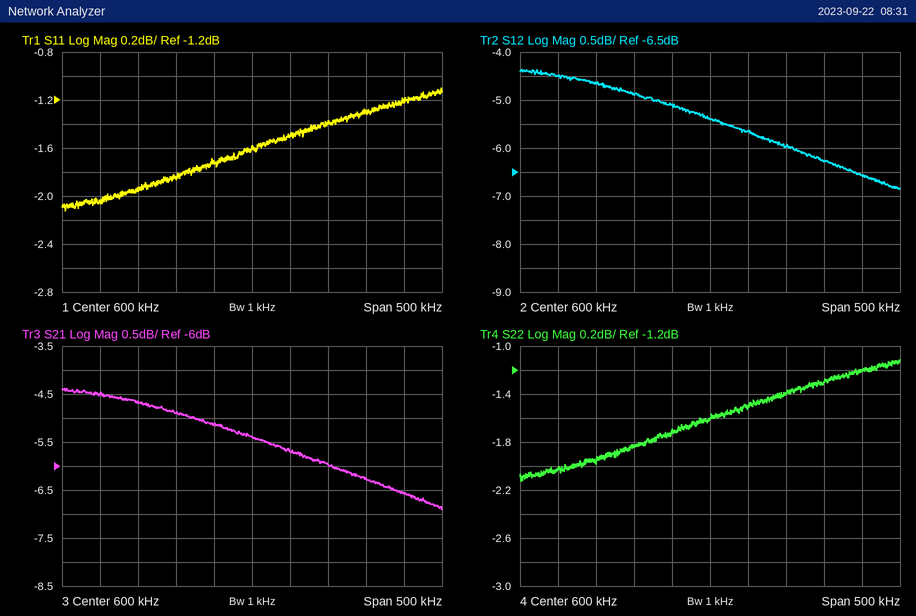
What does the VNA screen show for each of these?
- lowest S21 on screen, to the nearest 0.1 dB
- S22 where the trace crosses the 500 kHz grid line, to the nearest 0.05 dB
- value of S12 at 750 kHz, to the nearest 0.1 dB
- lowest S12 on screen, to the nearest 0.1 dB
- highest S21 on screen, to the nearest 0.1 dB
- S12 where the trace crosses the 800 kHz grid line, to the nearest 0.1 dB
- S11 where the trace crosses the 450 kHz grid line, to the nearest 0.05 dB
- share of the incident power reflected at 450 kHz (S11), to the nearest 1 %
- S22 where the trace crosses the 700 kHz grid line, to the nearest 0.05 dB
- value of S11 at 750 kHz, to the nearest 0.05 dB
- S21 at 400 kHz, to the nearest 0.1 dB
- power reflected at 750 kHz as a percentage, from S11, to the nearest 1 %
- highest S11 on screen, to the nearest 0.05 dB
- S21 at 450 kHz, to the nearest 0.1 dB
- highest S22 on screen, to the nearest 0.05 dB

-6.9 dB
-1.85 dB
-6.3 dB
-6.9 dB
-4.4 dB
-6.6 dB
-1.95 dB
64 %
-1.40 dB
-1.30 dB
-4.5 dB
74 %
-1.10 dB
-4.7 dB
-1.10 dB
